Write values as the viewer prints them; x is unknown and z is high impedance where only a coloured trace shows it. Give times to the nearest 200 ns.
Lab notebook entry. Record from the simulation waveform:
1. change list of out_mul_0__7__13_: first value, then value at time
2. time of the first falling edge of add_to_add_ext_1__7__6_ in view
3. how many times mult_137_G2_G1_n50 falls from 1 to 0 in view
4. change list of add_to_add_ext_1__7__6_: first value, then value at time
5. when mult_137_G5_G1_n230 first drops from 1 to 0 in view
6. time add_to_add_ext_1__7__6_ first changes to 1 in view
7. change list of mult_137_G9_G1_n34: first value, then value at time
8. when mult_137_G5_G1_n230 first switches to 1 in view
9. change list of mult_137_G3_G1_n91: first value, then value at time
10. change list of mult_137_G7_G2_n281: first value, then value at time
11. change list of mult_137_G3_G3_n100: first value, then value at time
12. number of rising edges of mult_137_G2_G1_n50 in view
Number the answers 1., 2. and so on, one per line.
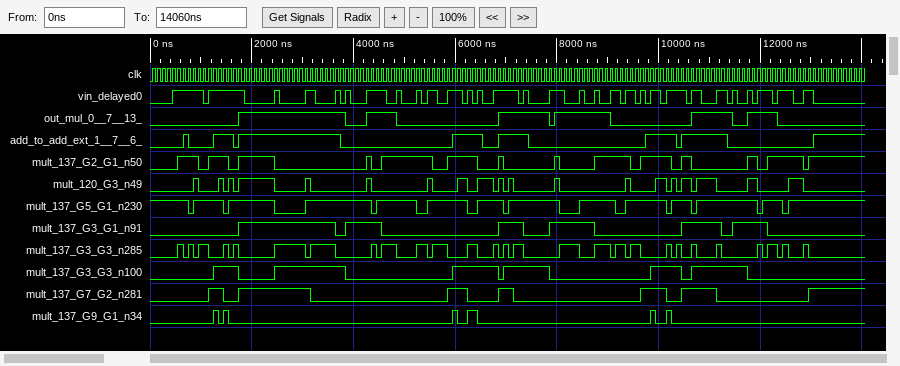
1. 0, 1 at 1800 ns, 0 at 3800 ns, 1 at 4200 ns, 0 at 4800 ns, 1 at 6800 ns, 0 at 7800 ns, 1 at 8000 ns, 0 at 9000 ns, 1 at 10600 ns, 0 at 11400 ns, 1 at 11800 ns, 0 at 12400 ns
2. 800 ns
3. 13
4. 0, 1 at 600 ns, 0 at 800 ns, 1 at 1200 ns, 0 at 1600 ns, 1 at 1800 ns, 0 at 3800 ns, 1 at 6000 ns, 0 at 6600 ns, 1 at 6800 ns, 0 at 7400 ns, 1 at 9800 ns, 0 at 10400 ns, 1 at 10400 ns, 0 at 11400 ns, 1 at 13000 ns
5. 800 ns
6. 600 ns
7. 0, 1 at 1200 ns, 0 at 1400 ns, 1 at 1400 ns, 0 at 1600 ns, 1 at 6000 ns, 0 at 6000 ns, 1 at 6200 ns, 0 at 6400 ns, 1 at 9800 ns, 0 at 10000 ns, 1 at 10200 ns, 0 at 10200 ns
8. 800 ns
9. 0, 1 at 1800 ns, 0 at 3600 ns, 1 at 3800 ns, 0 at 4600 ns, 1 at 6800 ns, 0 at 7400 ns, 1 at 7800 ns, 0 at 8800 ns, 1 at 10400 ns, 0 at 11200 ns, 1 at 11400 ns, 0 at 12200 ns
10. 0, 1 at 1200 ns, 0 at 1400 ns, 1 at 1800 ns, 0 at 3200 ns, 1 at 5800 ns, 0 at 6200 ns, 1 at 6800 ns, 0 at 7200 ns, 1 at 9600 ns, 0 at 10200 ns, 1 at 10400 ns, 0 at 11200 ns, 1 at 13000 ns
11. 0, 1 at 1200 ns, 0 at 1800 ns, 1 at 2400 ns, 0 at 3800 ns, 1 at 6000 ns, 0 at 6800 ns, 1 at 7000 ns, 0 at 7800 ns, 1 at 9800 ns, 0 at 10400 ns, 1 at 10600 ns, 0 at 11800 ns
12. 14
